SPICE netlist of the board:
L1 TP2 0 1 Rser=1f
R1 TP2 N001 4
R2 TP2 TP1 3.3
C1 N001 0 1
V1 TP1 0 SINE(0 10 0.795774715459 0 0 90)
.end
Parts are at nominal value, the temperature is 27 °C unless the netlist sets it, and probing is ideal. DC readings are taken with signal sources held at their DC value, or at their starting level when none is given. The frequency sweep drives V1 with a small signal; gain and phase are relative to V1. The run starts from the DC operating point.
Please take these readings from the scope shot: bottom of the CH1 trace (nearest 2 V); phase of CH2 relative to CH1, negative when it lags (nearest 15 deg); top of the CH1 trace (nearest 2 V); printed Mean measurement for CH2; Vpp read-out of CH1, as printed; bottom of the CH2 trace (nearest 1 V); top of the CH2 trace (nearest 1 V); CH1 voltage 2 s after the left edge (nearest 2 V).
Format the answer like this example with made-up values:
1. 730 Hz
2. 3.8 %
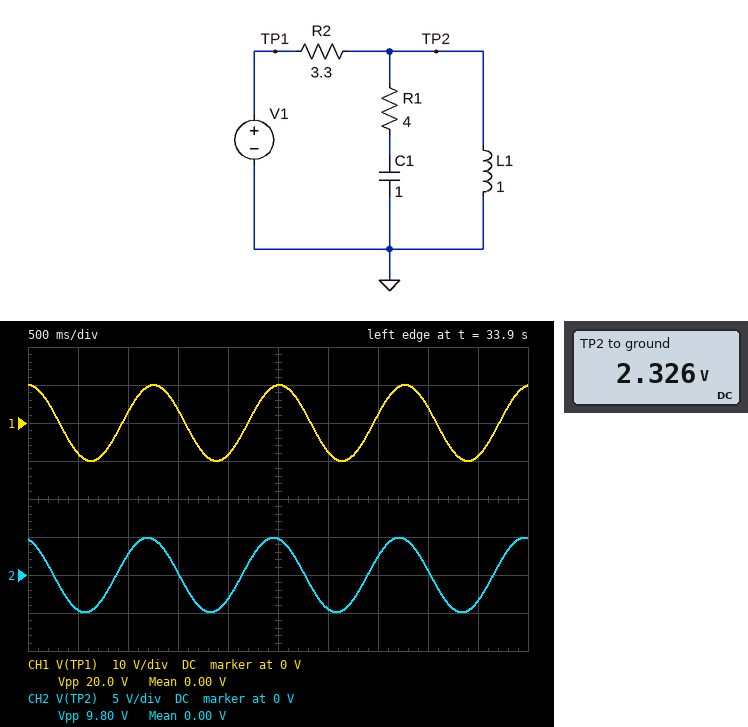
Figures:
1. -10 V
2. 15 deg
3. 10 V
4. 0.00 V
5. 20.0 V
6. -5 V
7. 5 V
8. -8 V
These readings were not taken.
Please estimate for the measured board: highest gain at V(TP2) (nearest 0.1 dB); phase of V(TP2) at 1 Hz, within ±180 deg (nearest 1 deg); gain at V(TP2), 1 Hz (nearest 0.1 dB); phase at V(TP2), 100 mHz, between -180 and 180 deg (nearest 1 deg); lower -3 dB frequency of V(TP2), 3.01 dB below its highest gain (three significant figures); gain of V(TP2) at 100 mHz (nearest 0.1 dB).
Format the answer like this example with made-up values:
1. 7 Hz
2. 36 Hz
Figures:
1. -5.2 dB
2. 14 deg
3. -5.9 dB
4. 16 deg
5. 370 mHz
6. -12.6 dB
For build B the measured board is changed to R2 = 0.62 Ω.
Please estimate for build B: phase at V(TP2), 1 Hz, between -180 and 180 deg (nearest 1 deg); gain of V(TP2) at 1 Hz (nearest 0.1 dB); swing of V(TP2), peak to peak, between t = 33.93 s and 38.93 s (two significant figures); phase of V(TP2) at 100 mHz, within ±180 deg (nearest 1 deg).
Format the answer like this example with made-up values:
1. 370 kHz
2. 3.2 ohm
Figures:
1. 4 deg
2. -1.4 dB
3. 17 V
4. 8 deg
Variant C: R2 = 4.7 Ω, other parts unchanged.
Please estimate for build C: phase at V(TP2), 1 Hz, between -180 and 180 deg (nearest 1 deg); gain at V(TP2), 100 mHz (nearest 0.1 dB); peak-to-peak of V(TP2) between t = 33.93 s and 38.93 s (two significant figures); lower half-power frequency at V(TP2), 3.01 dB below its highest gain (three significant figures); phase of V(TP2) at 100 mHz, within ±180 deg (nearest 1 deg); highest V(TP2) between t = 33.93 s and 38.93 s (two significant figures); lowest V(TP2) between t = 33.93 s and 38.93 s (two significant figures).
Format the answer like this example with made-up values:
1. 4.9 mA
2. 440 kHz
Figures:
1. 17 deg
2. -15.0 dB
3. 8.0 V
4. 431 mHz
5. 18 deg
6. 4.0 V
7. -4.0 V
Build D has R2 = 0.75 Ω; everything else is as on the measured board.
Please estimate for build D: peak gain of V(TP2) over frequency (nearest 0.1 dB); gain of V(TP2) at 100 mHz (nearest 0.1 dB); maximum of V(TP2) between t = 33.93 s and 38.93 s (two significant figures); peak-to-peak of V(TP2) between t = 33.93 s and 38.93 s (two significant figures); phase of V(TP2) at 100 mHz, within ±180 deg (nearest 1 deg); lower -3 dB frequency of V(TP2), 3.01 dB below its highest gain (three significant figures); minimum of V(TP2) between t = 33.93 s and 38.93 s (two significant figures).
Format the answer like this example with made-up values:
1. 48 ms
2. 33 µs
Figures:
1. -1.5 dB
2. -4.7 dB
3. 8.2 V
4. 16 V
5. 9 deg
6. 118 mHz
7. -8.2 V
